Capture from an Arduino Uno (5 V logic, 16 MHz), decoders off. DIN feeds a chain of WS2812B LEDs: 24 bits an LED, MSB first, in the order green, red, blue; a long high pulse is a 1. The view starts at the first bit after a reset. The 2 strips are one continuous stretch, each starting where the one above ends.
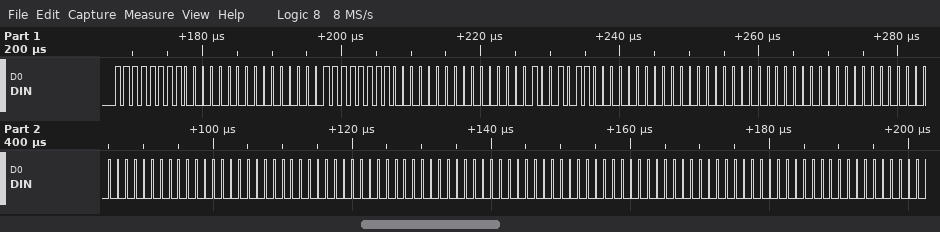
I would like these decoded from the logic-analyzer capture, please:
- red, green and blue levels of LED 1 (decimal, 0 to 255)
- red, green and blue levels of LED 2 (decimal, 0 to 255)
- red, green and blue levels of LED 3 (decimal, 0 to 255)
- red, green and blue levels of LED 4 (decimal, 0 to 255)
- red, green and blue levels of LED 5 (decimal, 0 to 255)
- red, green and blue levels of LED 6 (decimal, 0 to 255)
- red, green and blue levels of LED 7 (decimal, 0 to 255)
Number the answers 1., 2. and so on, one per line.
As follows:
1. 0, 255, 0
2. 0, 255, 0
3. 0, 150, 0
4. 0, 0, 0
5. 0, 0, 0
6. 0, 0, 0
7. 0, 0, 0
